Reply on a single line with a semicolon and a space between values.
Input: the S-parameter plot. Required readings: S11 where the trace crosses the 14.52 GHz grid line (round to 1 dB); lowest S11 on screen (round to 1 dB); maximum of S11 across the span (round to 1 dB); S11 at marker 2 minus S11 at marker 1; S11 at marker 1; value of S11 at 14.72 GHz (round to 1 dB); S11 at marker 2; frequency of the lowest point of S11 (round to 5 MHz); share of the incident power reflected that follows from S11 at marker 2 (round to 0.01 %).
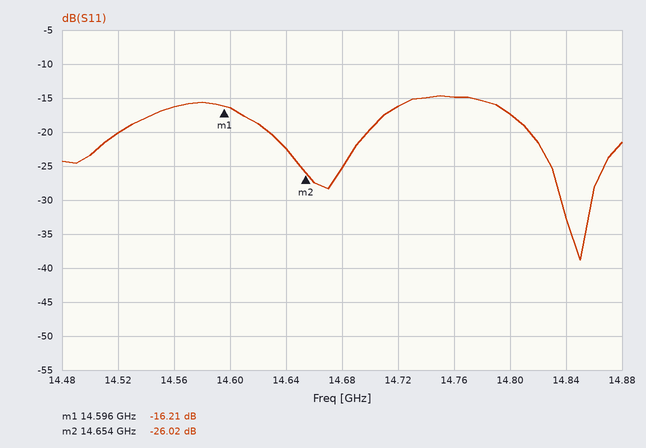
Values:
-20 dB; -39 dB; -15 dB; -9.81 dB; -16.21 dB; -16 dB; -26.02 dB; 14.850 GHz; 0.25 %
